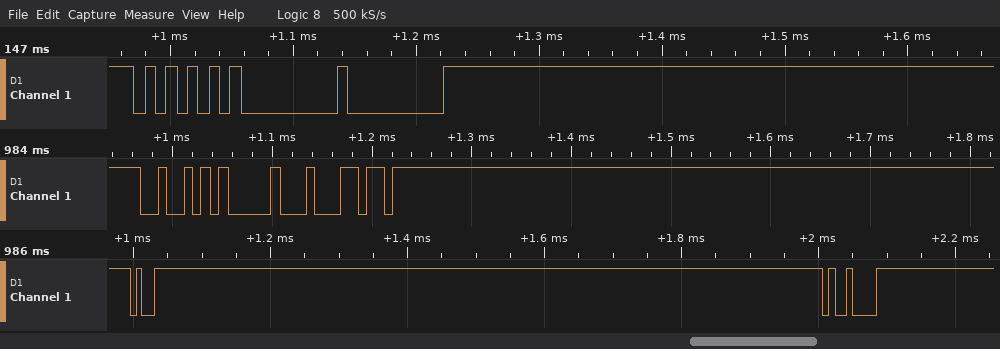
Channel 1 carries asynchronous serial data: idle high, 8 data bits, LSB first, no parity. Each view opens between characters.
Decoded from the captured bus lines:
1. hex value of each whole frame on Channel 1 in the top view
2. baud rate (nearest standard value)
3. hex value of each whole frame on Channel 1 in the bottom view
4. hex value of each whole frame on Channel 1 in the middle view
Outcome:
55, 00, 00
115200 baud
F9, 09
52, 10, 6C
